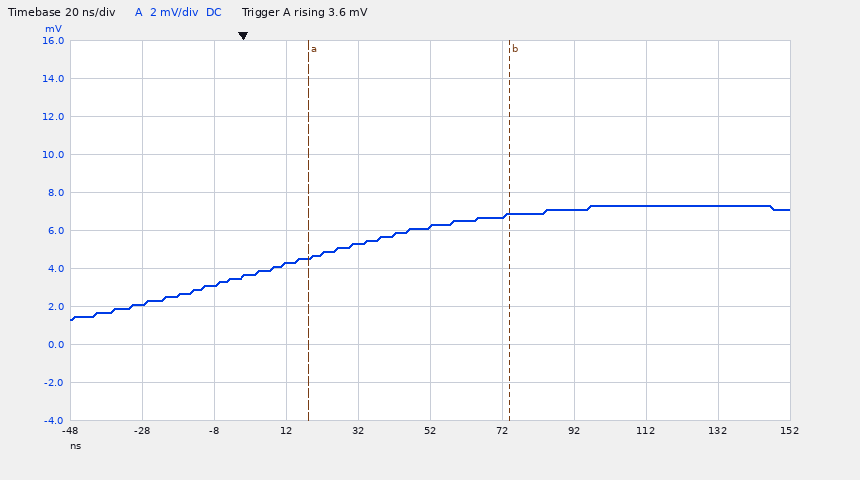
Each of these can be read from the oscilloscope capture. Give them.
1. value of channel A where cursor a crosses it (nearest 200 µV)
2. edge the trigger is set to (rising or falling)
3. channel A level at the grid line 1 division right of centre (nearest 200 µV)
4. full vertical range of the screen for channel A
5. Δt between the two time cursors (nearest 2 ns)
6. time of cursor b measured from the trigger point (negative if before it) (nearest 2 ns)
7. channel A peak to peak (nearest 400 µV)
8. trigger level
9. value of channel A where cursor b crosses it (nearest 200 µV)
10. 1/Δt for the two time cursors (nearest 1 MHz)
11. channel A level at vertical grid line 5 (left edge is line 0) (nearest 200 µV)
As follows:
4.6 mV
rising
6.8 mV
20 mV
56 ns
+74 ns
6.0 mV
3.6 mV
6.8 mV
18 MHz
6.2 mV
